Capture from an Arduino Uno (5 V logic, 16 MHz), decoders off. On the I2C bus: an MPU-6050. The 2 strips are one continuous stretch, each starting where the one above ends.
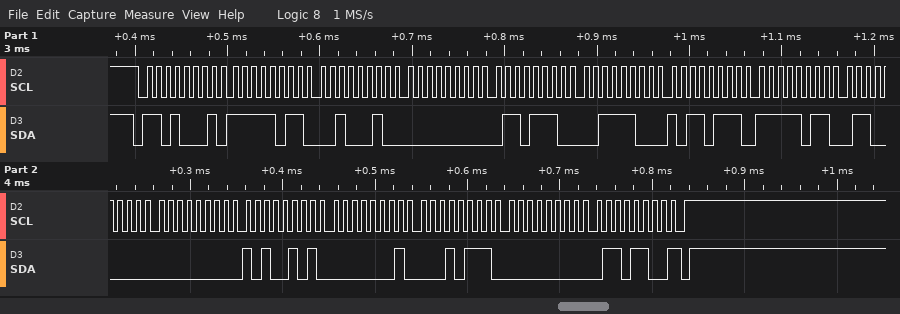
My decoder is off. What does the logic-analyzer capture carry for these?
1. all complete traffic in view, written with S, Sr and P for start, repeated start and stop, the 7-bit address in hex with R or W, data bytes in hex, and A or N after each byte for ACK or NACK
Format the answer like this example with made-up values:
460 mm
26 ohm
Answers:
S 68R A FB A 22 A 00 A 6E A 3C A B7 A FB A 60 A 00 A A5 A 01 A 17 A 00 A 6C N P
